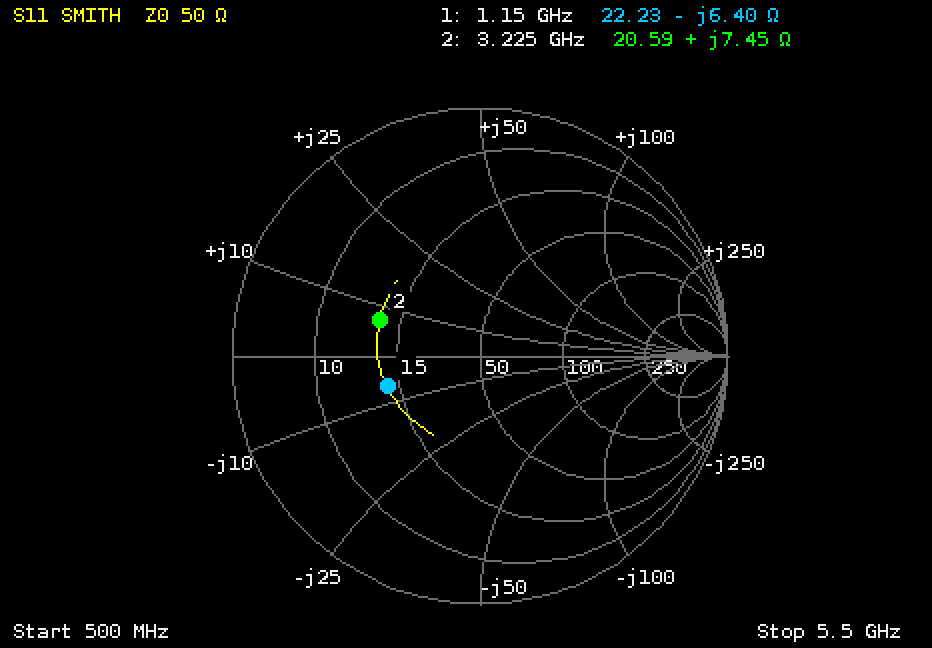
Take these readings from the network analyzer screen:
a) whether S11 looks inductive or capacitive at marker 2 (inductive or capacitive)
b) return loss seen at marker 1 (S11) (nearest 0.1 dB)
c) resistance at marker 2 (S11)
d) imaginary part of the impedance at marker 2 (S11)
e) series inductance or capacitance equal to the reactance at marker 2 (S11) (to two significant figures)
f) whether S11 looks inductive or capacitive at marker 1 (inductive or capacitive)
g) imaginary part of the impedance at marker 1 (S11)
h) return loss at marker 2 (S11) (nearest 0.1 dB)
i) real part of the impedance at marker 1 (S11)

inductive
8.1 dB
20.59 Ω
+7.45 Ω
370 pH
capacitive
-6.40 Ω
7.4 dB
22.23 Ω
